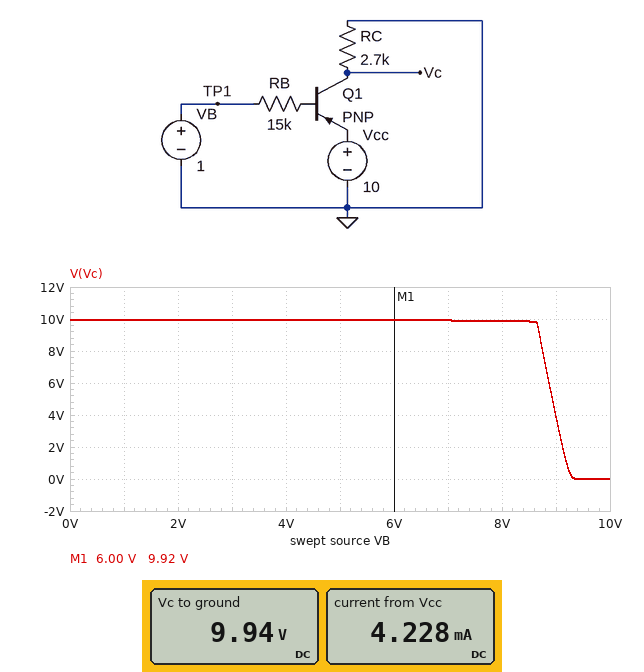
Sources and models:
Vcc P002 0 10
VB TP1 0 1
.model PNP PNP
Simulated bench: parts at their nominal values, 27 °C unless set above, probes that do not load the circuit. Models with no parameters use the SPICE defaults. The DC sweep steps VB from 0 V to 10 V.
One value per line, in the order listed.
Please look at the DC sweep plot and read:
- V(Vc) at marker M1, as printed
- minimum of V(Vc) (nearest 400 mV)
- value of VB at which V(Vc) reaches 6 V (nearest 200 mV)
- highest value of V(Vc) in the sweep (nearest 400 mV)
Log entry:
9.92 V
0 V
8.8 V
10.0 V
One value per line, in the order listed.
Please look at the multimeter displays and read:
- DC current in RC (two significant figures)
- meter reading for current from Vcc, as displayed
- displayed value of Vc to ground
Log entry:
3.7 mA
4.228 mA
9.94 V
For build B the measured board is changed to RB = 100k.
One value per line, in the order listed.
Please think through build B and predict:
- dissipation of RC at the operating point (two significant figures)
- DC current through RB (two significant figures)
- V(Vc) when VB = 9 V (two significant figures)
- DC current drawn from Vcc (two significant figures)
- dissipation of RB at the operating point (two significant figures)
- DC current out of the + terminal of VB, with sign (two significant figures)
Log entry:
36 mW
82 µA
700 mV
3.7 mA
670 µW
-82 µA
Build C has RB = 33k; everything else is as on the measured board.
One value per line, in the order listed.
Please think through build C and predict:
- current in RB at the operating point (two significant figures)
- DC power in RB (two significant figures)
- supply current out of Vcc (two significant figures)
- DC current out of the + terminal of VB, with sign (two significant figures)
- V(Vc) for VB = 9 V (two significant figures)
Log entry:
250 µA
2.0 mW
3.9 mA
-250 µA
1.9 V
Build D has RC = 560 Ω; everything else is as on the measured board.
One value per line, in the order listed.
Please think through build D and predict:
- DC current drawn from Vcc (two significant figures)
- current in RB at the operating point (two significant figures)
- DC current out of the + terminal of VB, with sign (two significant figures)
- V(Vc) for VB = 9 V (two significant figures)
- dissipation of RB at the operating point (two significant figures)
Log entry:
18 mA
540 µA
-540 µA
810 mV
4.4 mW
